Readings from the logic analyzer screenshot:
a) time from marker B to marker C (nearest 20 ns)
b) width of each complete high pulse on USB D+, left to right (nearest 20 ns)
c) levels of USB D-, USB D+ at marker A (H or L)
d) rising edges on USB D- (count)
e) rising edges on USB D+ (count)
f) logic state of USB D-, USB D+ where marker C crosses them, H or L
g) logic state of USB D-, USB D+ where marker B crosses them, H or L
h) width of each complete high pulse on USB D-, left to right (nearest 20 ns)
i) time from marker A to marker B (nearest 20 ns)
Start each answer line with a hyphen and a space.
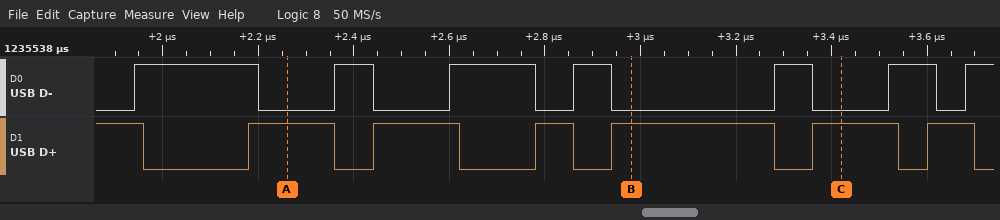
- 440 ns
- 180 ns, 180 ns, 80 ns, 340 ns, 180 ns, 100 ns
- USB D-=L, USB D+=H
- 7
- 6
- USB D-=L, USB D+=H
- USB D-=L, USB D+=H
- 260 ns, 80 ns, 180 ns, 80 ns, 80 ns, 100 ns
- 720 ns
